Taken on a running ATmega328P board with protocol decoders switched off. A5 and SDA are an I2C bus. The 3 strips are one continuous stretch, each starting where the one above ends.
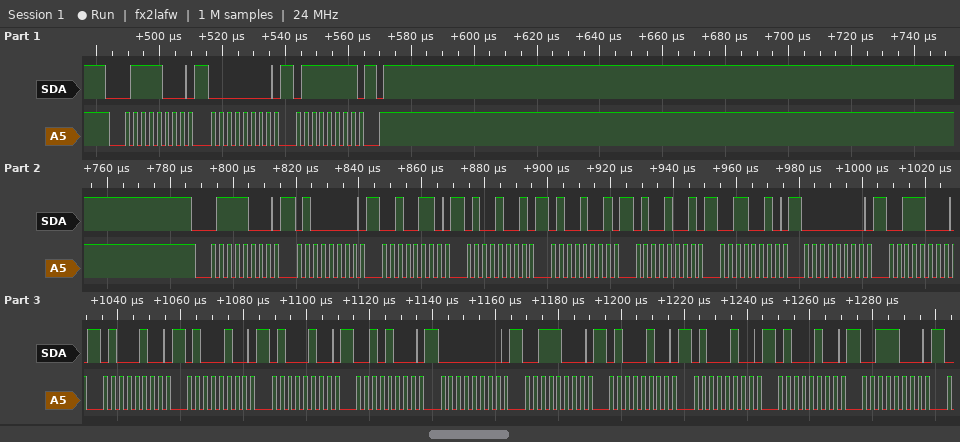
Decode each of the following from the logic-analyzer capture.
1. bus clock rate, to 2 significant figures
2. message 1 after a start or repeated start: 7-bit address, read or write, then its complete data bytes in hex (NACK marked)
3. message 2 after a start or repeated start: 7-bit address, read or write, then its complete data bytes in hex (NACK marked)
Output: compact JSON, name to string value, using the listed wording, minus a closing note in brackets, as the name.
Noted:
{"bus clock rate, to 2 significant figures": "400 kHz", "message 1 after a start or repeated start: 7-bit address, read or write, then its complete data bytes in hex": "0x3C write: 00 7F", "message 2 after a start or repeated start: 7-bit address, read or write, then its complete data bytes in hex": "0x3C write: 40 26 49 49 49 32 00 38 44 44 44 28 00 38 44 44 44 38"}
